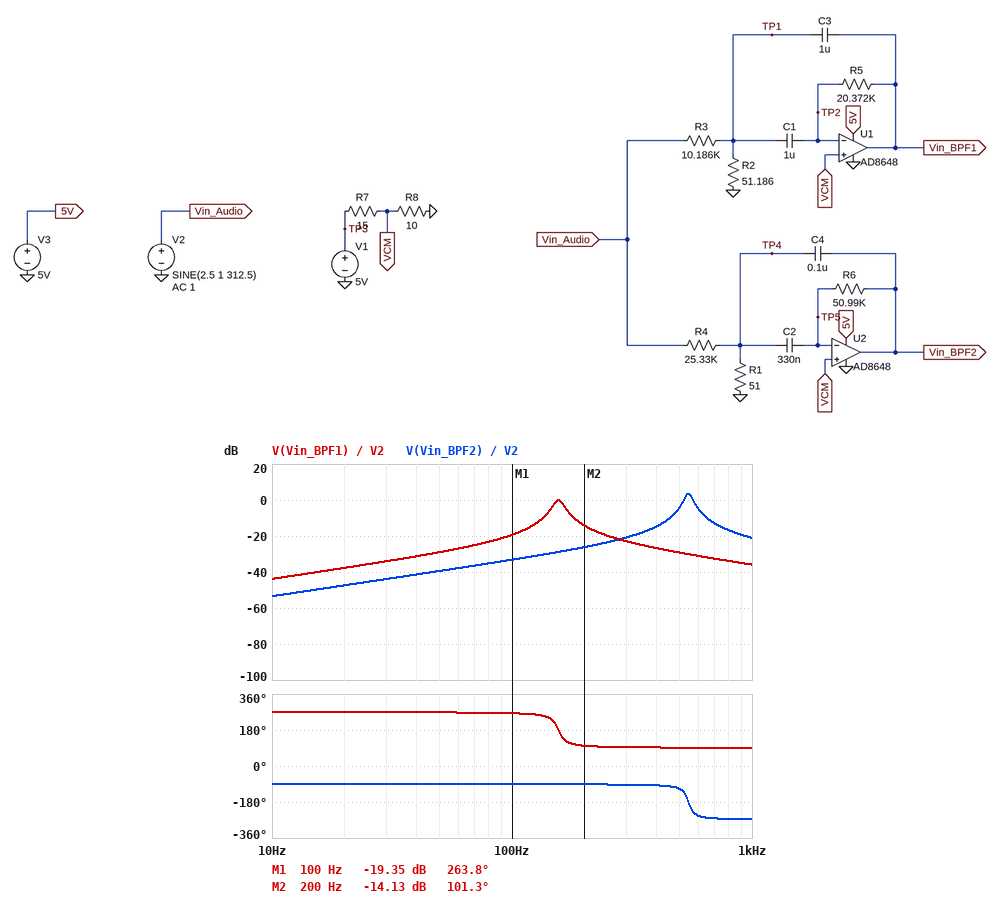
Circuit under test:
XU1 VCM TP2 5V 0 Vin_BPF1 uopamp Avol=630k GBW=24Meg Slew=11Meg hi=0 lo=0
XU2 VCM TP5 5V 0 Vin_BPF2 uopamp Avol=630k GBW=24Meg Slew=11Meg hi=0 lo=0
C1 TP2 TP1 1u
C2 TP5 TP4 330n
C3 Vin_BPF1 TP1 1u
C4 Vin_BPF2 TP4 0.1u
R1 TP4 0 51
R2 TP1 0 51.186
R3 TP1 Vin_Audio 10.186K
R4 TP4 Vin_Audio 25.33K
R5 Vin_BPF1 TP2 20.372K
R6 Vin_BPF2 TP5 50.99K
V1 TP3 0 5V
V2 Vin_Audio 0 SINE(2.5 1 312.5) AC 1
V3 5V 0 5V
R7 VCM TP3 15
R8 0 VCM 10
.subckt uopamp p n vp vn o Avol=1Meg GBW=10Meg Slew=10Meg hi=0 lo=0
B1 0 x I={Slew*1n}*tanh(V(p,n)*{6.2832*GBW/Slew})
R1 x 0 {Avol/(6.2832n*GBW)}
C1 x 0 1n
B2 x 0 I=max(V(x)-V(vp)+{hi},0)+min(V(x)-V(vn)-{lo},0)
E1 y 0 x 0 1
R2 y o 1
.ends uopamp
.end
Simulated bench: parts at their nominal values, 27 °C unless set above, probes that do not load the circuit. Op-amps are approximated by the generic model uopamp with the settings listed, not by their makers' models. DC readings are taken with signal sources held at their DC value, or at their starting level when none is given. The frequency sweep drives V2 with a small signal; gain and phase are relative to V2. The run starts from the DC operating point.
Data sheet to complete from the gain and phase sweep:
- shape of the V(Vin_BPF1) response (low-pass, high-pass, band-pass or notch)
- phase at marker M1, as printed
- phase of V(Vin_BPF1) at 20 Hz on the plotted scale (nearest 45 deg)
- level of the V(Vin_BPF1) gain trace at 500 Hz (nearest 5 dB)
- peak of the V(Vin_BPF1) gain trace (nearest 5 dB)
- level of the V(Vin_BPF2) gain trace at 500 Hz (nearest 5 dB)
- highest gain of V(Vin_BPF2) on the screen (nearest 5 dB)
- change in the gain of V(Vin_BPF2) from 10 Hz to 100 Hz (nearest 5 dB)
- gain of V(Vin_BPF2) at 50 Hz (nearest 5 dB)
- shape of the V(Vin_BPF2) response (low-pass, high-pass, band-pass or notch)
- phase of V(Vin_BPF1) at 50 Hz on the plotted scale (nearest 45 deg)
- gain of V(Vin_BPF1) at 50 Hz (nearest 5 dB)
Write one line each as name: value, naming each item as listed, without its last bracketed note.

shape of the V(Vin_BPF1) response: band-pass
phase at marker M1, as printed: 263.8 deg
phase of V(Vin_BPF1) at 20 Hz on the plotted scale: 270 deg
level of the V(Vin_BPF1) gain trace at 500 Hz: -30 dB
peak of the V(Vin_BPF1) gain trace: 0 dB
level of the V(Vin_BPF2) gain trace at 500 Hz: -5 dB
highest gain of V(Vin_BPF2) on the screen: 5 dB
change in the gain of V(Vin_BPF2) from 10 Hz to 100 Hz: 20 dB
gain of V(Vin_BPF2) at 50 Hz: -40 dB
shape of the V(Vin_BPF2) response: band-pass
phase of V(Vin_BPF1) at 50 Hz on the plotted scale: 270 deg
gain of V(Vin_BPF1) at 50 Hz: -30 dB
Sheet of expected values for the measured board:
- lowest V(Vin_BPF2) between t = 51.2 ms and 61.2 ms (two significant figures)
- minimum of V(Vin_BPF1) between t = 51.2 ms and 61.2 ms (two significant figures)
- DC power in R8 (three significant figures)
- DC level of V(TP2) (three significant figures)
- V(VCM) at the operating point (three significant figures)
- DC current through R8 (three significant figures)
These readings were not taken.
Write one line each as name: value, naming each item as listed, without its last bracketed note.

lowest V(Vin_BPF2) between t = 51.2 ms and 61.2 ms: 1.9 V
minimum of V(Vin_BPF1) between t = 51.2 ms and 61.2 ms: 1.9 V
DC power in R8: 400 mW
DC level of V(TP2): 2.00 V
V(VCM) at the operating point: 2.00 V
DC current through R8: 200 mA
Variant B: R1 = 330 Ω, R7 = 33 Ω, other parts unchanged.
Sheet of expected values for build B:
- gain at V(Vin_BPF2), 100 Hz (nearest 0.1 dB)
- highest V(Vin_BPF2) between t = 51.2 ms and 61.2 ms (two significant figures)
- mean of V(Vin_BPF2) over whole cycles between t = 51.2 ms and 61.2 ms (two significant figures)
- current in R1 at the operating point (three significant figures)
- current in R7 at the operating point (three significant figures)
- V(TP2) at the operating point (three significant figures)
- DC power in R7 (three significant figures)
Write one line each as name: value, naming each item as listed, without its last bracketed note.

gain at V(Vin_BPF2), 100 Hz: -15.3 dB
highest V(Vin_BPF2) between t = 51.2 ms and 61.2 ms: 1.5 V
mean of V(Vin_BPF2) over whole cycles between t = 51.2 ms and 61.2 ms: 1.2 V
current in R1 at the operating point: 97.4 µA
current in R7 at the operating point: 116 mA
V(TP2) at the operating point: 1.16 V
DC power in R7: 446 mW
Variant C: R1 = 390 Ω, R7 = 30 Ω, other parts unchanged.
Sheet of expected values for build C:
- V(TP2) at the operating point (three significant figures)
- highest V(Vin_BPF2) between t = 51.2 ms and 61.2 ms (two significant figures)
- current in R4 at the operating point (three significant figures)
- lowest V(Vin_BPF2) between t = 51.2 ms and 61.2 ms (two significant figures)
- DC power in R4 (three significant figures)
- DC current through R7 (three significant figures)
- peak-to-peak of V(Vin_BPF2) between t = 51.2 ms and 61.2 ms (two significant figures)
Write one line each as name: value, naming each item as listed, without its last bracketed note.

V(TP2) at the operating point: 1.25 V
highest V(Vin_BPF2) between t = 51.2 ms and 61.2 ms: 1.6 V
current in R4 at the operating point: 97.2 µA
lowest V(Vin_BPF2) between t = 51.2 ms and 61.2 ms: 920 mV
DC power in R4: 239 µW
DC current through R7: 125 mA
peak-to-peak of V(Vin_BPF2) between t = 51.2 ms and 61.2 ms: 660 mV
